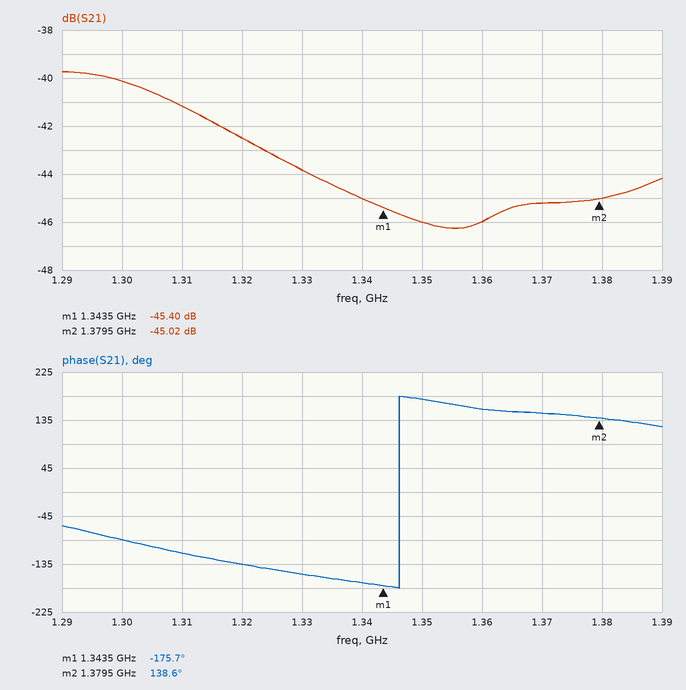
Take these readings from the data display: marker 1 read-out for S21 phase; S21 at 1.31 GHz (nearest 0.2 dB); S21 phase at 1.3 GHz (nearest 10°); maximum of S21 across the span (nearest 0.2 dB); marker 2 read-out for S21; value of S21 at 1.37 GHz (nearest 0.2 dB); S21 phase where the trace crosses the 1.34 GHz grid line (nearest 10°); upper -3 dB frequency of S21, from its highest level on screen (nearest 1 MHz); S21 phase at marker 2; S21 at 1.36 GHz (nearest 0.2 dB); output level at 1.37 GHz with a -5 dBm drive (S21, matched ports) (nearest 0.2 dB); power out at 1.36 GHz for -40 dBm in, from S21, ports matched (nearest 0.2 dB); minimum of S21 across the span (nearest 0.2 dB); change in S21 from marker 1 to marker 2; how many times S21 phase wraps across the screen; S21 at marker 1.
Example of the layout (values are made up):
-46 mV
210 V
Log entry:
-175.7°
-41.2 dB
-90°
-39.8 dB
-45.02 dB
-45.2 dB
-170°
1.322 GHz
138.6°
-46.0 dB
-50.2 dBm
-86.0 dBm
-46.2 dB
0.38 dB
1
-45.40 dB
